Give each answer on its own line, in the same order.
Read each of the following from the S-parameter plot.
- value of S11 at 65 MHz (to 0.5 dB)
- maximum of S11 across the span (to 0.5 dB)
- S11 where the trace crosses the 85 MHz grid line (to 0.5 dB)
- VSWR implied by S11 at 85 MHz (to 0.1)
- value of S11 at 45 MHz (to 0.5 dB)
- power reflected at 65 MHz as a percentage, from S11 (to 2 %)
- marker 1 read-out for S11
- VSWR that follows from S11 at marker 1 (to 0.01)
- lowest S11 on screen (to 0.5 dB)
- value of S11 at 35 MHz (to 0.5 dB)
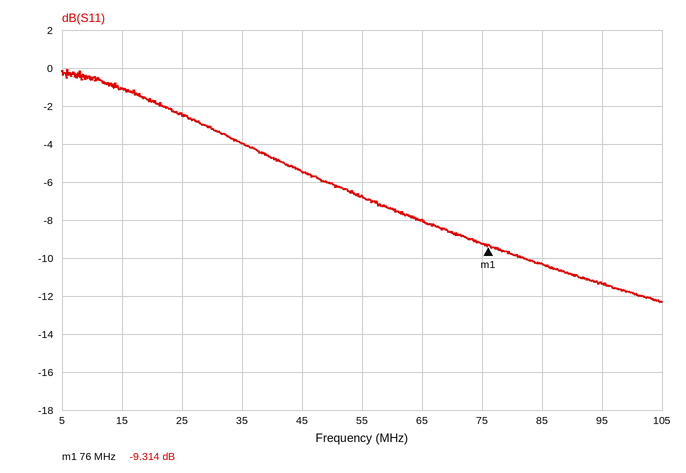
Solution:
-8.0 dB
0.0 dB
-10.5 dB
1.9
-5.5 dB
16 %
-9.314 dB
2.04
-12.5 dB
-4.0 dB
